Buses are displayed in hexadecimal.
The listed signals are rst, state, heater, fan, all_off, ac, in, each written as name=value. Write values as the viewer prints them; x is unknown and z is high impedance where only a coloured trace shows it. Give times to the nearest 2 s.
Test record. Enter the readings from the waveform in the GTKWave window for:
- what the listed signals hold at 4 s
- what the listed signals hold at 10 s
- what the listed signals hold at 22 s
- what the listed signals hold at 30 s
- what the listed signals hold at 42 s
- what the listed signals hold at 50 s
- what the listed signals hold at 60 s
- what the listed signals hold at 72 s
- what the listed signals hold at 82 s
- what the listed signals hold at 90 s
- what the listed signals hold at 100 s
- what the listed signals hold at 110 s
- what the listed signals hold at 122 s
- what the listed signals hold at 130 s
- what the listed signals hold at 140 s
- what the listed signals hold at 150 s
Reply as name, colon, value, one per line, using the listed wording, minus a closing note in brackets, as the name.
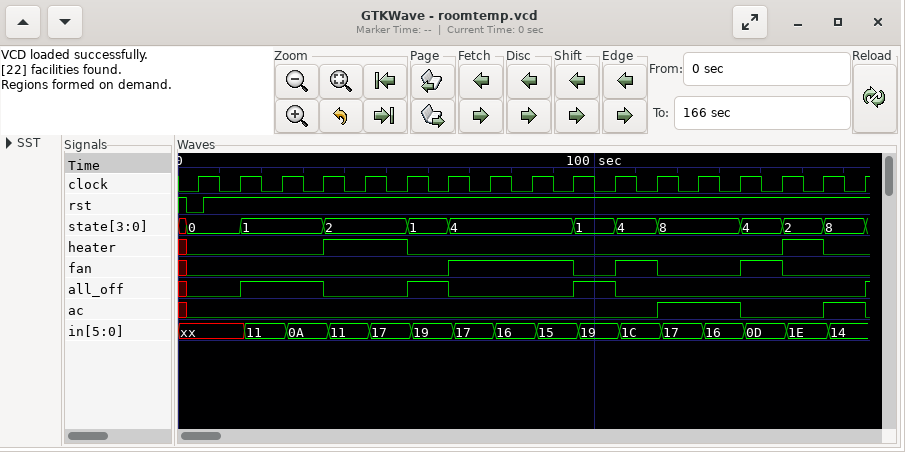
what the listed signals hold at 4 s: rst=0, state=0, heater=0, fan=0, all_off=0, ac=0, in=xx
what the listed signals hold at 10 s: rst=1, state=0, heater=0, fan=0, all_off=0, ac=0, in=xx
what the listed signals hold at 22 s: rst=1, state=1, heater=0, fan=0, all_off=1, ac=0, in=11
what the listed signals hold at 30 s: rst=1, state=1, heater=0, fan=0, all_off=1, ac=0, in=0A
what the listed signals hold at 42 s: rst=1, state=2, heater=1, fan=0, all_off=0, ac=0, in=11
what the listed signals hold at 50 s: rst=1, state=2, heater=1, fan=0, all_off=0, ac=0, in=17
what the listed signals hold at 60 s: rst=1, state=1, heater=0, fan=0, all_off=1, ac=0, in=19
what the listed signals hold at 72 s: rst=1, state=4, heater=0, fan=1, all_off=0, ac=0, in=17
what the listed signals hold at 82 s: rst=1, state=4, heater=0, fan=1, all_off=0, ac=0, in=16
what the listed signals hold at 90 s: rst=1, state=4, heater=0, fan=1, all_off=0, ac=0, in=15
what the listed signals hold at 100 s: rst=1, state=1, heater=0, fan=0, all_off=1, ac=0, in=19
what the listed signals hold at 110 s: rst=1, state=4, heater=0, fan=1, all_off=0, ac=0, in=1C
what the listed signals hold at 122 s: rst=1, state=8, heater=0, fan=0, all_off=0, ac=1, in=17
what the listed signals hold at 130 s: rst=1, state=8, heater=0, fan=0, all_off=0, ac=1, in=16
what the listed signals hold at 140 s: rst=1, state=4, heater=0, fan=1, all_off=0, ac=0, in=0D
what the listed signals hold at 150 s: rst=1, state=2, heater=1, fan=0, all_off=0, ac=0, in=1E
